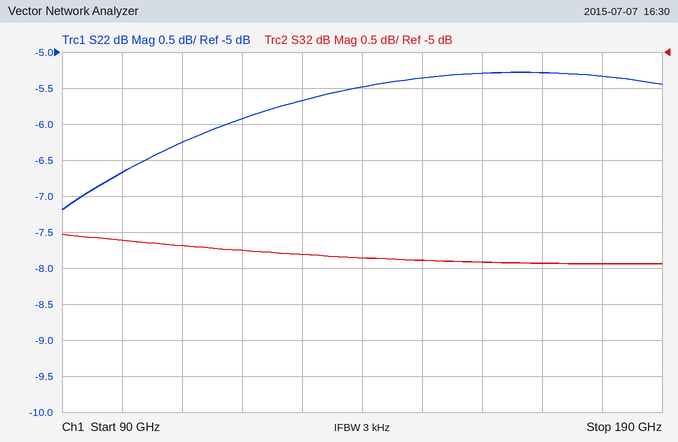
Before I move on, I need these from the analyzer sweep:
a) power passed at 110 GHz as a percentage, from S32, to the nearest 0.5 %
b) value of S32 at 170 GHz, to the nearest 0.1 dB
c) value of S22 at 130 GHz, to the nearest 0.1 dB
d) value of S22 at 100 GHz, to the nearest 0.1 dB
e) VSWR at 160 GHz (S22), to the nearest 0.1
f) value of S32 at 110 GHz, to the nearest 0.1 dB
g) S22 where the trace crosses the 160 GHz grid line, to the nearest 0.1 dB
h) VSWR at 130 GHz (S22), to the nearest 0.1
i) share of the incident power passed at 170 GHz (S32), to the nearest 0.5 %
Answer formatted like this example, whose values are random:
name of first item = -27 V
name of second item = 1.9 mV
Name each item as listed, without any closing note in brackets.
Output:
power passed at 110 GHz as a percentage, from S32, to the nearest 0.5 % = 17.0 %
value of S32 at 170 GHz, to the nearest 0.1 dB = -7.9 dB
value of S22 at 130 GHz, to the nearest 0.1 dB = -5.7 dB
value of S22 at 100 GHz, to the nearest 0.1 dB = -6.7 dB
VSWR at 160 GHz (S22), to the nearest 0.1 = 3.4
value of S32 at 110 GHz, to the nearest 0.1 dB = -7.7 dB
S22 where the trace crosses the 160 GHz grid line, to the nearest 0.1 dB = -5.3 dB
VSWR at 130 GHz (S22), to the nearest 0.1 = 3.2
share of the incident power passed at 170 GHz (S32), to the nearest 0.5 % = 16.0 %
